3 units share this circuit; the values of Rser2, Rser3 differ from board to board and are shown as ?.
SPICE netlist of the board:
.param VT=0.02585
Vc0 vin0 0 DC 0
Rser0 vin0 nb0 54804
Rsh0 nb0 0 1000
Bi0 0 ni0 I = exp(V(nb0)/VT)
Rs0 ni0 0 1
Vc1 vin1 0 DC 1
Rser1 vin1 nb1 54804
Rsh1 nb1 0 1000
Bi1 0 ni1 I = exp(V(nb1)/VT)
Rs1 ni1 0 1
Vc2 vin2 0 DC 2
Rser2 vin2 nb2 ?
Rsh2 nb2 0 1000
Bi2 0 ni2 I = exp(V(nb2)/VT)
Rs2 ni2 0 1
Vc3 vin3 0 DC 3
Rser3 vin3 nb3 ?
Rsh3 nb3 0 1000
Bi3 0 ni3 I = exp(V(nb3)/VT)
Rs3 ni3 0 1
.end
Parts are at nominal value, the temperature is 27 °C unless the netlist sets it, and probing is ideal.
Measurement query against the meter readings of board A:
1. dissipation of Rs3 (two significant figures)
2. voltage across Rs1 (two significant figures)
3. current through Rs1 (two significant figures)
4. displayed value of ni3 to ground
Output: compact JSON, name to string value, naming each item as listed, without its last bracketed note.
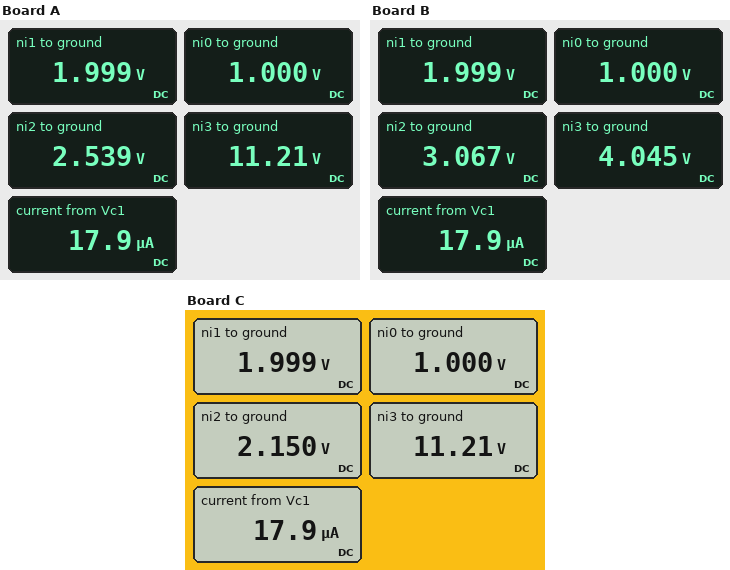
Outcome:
{"dissipation of Rs3": "130 W", "voltage across Rs1": "2.0 V", "current through Rs1": "2.0 A", "displayed value of ni3 to ground": "11.21 V"}
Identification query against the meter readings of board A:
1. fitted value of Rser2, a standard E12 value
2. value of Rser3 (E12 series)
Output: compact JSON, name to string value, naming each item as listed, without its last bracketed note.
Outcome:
{"fitted value of Rser2, a standard E12 value": "82 kΩ", "value of Rser3": "47 kΩ"}
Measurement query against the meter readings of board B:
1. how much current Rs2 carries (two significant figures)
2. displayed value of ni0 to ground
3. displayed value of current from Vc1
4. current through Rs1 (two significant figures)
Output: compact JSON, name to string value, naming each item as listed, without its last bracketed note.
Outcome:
{"how much current Rs2 carries": "3.1 A", "displayed value of ni0 to ground": "1.000 V", "displayed value of current from Vc1": "17.9 µA", "current through Rs1": "2.0 A"}
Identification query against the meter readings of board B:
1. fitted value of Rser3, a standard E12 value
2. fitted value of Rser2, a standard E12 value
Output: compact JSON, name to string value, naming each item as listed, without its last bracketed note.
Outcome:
{"fitted value of Rser3, a standard E12 value": "82 kΩ", "fitted value of Rser2, a standard E12 value": "68 kΩ"}
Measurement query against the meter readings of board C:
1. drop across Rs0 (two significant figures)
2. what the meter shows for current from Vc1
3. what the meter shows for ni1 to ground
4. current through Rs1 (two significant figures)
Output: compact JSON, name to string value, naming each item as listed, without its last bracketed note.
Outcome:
{"drop across Rs0": "1.0 V", "what the meter shows for current from Vc1": "17.9 µA", "what the meter shows for ni1 to ground": "1.999 V", "current through Rs1": "2.0 A"}
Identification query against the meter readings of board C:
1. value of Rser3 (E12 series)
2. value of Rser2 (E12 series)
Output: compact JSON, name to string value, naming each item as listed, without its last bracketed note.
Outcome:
{"value of Rser3": "47 kΩ", "value of Rser2": "100 kΩ"}
